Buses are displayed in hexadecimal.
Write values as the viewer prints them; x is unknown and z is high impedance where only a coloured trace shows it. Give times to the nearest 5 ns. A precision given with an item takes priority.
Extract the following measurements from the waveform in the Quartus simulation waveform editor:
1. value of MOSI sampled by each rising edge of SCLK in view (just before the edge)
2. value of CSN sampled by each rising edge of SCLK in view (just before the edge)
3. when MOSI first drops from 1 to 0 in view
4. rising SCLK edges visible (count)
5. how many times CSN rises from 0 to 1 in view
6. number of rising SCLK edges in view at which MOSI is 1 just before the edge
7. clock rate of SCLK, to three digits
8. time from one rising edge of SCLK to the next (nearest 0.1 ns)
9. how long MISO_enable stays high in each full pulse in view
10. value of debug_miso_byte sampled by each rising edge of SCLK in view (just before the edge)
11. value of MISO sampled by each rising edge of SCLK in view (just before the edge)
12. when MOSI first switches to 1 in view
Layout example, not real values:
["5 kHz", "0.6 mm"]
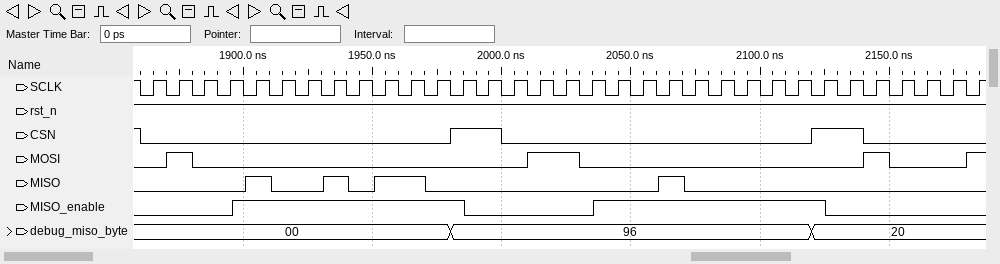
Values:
["0 1 0 0 0 0 0 0 0 0 0 0 0 0 0 1 1 0 0 0 0 0 0 0 0 0 0 0 1 0 0 0 1", "0 0 0 0 0 0 0 0 0 0 0 0 1 1 0 0 0 0 0 0 0 0 0 0 0 0 1 1 0 0 0 0 0", "1880 ns", "33", "2", "5", "100 MHz", "10 ns", "90 ns, 90 ns", "00, 00, 00, 00, 00, 00, 00, 00, 00, 00, 00, 00, 96, 96, 96, 96, 96, 96, 96, 96, 96, 96, 96, 96, 96, 96, 20, 20, 20, 20, 20, 20, 20", "0 0 0 0 1 0 0 1 0 1 1 0 0 0 0 0 0 0 0 0 1 0 0 0 0 0 0 0 0 0 0 0 0", "1870 ns"]
